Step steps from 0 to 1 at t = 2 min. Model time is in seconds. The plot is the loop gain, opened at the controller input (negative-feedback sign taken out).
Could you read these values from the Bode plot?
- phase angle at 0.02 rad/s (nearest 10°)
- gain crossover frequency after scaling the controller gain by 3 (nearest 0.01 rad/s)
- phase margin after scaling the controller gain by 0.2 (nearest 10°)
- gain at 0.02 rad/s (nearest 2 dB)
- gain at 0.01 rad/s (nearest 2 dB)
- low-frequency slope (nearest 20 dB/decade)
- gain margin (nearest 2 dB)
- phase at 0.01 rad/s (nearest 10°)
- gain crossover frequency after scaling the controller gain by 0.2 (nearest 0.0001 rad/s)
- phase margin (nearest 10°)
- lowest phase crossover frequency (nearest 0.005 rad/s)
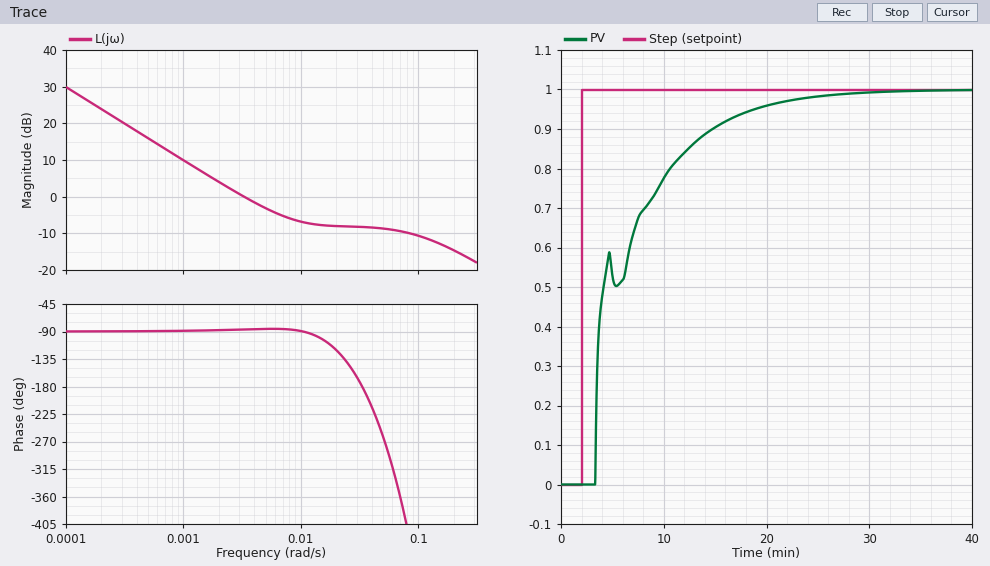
-120°
0.07 rad/s
90°
-8 dB
-6 dB
-20 dB/decade
8 dB
-90°
0.0006 rad/s
90°
0.035 rad/s
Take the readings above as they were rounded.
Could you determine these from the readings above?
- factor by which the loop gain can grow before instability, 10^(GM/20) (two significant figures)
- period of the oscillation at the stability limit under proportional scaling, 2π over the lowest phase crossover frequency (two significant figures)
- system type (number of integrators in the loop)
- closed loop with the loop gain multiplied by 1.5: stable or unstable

2.5
180 s
1
stable
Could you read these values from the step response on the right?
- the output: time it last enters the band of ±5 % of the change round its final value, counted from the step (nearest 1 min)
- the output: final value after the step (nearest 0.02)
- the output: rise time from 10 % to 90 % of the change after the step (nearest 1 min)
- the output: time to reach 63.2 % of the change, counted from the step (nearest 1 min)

17 min
1.00
11 min
5 min
